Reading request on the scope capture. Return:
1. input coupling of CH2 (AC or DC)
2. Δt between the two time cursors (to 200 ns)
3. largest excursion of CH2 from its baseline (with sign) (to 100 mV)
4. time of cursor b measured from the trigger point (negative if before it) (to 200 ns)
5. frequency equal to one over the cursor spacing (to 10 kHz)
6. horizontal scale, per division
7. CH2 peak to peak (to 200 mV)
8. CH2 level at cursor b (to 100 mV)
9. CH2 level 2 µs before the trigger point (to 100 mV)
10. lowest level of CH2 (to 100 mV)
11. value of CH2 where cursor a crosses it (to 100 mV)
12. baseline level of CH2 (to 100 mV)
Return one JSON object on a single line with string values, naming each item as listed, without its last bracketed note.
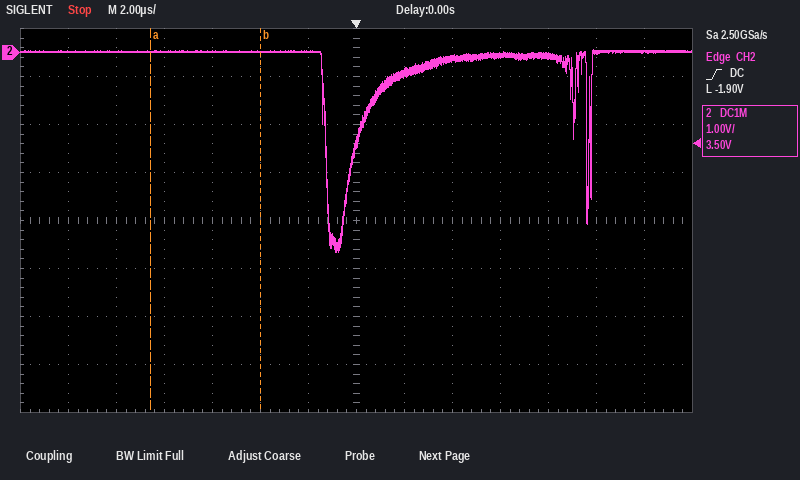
{"input coupling of CH2": "DC", "Δt between the two time cursors": "4.6 µs", "largest excursion of CH2 from its baseline (with sign)": "-4.2 V", "time of cursor b measured from the trigger point (negative if before it)": "-4.0 µs", "frequency equal to one over the cursor spacing": "220 kHz", "horizontal scale, per division": "2 µs", "CH2 peak to peak": "4.2 V", "CH2 level at cursor b": "0.0 V", "CH2 level 2 µs before the trigger point": "0.0 V", "lowest level of CH2": "-4.2 V", "value of CH2 where cursor a crosses it": "0.0 V", "baseline level of CH2": "0.0 V"}
